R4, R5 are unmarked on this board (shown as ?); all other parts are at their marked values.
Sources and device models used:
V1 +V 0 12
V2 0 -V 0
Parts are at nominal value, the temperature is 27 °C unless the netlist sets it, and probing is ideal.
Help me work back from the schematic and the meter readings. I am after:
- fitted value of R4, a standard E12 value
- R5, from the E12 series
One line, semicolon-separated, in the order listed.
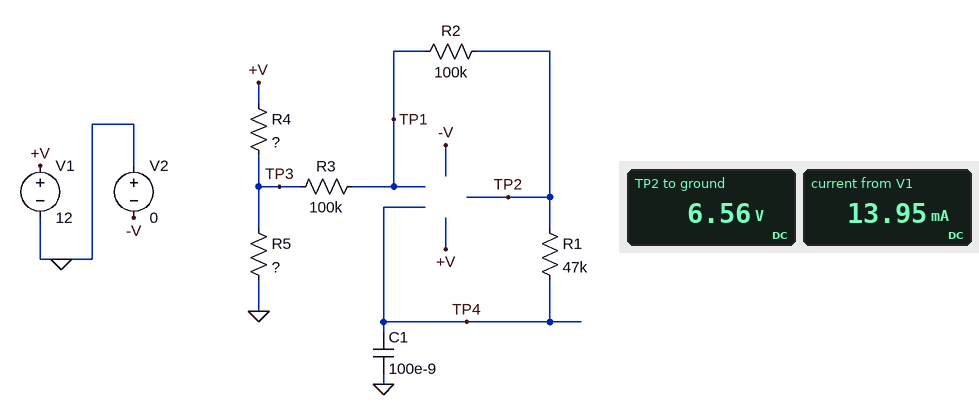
390 Ω; 470 Ω
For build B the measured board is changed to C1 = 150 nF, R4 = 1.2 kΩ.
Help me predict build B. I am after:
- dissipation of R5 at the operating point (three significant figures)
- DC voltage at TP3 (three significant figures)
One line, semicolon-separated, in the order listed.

24.3 mW; 3.38 V
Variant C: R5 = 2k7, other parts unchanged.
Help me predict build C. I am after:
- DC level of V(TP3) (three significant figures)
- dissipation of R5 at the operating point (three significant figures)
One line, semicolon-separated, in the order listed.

10.5 V; 40.7 mW
